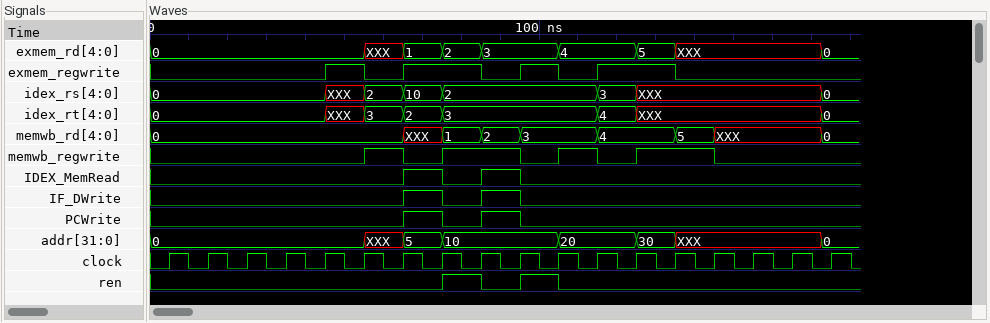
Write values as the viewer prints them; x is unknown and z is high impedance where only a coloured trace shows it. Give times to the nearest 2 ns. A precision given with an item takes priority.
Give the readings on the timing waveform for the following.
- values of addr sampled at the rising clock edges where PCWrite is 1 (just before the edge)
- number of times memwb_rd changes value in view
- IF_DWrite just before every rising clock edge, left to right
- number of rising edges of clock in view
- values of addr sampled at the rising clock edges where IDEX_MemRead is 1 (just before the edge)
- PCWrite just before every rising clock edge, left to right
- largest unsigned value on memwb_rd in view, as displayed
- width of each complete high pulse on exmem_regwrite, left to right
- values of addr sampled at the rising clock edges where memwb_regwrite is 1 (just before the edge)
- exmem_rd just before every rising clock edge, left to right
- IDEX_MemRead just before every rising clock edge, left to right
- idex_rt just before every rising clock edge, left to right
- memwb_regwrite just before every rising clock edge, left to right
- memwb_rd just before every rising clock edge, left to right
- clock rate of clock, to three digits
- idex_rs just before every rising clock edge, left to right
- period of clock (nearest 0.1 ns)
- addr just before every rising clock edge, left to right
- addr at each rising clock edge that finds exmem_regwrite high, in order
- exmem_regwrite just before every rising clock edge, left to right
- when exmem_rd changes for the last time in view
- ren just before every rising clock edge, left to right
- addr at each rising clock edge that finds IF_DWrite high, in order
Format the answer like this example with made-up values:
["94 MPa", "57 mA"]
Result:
["5, 10", "8", "0 0 0 0 0 0 0 1 0 1 0 0 0 0 0 0 0 0", "18", "5, 10", "0 0 0 0 0 0 0 1 0 1 0 0 0 0 0 0 0 0", "5", "10 ns, 20 ns, 10 ns, 20 ns", "XXX, 10, 10, 20, 30, XXX", "0, 0, 0, 0, 0, 0, XXX, 1, 2, 3, 3, 4, 4, 5, XXX, XXX, XXX, 0", "0 0 0 0 0 0 0 1 0 1 0 0 0 0 0 0 0 0", "0, 0, 0, 0, 0, XXX, 3, 2, 3, 3, 3, 3, 4, XXX, XXX, XXX, XXX, 0", "0 0 0 0 0 0 1 0 1 1 0 1 0 1 1 0 0 0", "0, 0, 0, 0, 0, 0, 0, XXX, 1, 2, 3, 3, 4, 4, 5, XXX, XXX, 0", "100 MHz", "0, 0, 0, 0, 0, XXX, 2, 10, 2, 2, 2, 2, 3, XXX, XXX, XXX, XXX, 0", "10 ns", "0, 0, 0, 0, 0, 0, XXX, 5, 10, 10, 10, 20, 20, 30, XXX, XXX, XXX, 0", "0, 5, 10, 10, 20, 30", "0 0 0 0 0 1 0 1 1 0 1 0 1 1 0 0 0 0", "172 ns", "0 0 0 0 0 0 0 0 1 0 1 0 0 0 0 0 0 0", "5, 10"]
